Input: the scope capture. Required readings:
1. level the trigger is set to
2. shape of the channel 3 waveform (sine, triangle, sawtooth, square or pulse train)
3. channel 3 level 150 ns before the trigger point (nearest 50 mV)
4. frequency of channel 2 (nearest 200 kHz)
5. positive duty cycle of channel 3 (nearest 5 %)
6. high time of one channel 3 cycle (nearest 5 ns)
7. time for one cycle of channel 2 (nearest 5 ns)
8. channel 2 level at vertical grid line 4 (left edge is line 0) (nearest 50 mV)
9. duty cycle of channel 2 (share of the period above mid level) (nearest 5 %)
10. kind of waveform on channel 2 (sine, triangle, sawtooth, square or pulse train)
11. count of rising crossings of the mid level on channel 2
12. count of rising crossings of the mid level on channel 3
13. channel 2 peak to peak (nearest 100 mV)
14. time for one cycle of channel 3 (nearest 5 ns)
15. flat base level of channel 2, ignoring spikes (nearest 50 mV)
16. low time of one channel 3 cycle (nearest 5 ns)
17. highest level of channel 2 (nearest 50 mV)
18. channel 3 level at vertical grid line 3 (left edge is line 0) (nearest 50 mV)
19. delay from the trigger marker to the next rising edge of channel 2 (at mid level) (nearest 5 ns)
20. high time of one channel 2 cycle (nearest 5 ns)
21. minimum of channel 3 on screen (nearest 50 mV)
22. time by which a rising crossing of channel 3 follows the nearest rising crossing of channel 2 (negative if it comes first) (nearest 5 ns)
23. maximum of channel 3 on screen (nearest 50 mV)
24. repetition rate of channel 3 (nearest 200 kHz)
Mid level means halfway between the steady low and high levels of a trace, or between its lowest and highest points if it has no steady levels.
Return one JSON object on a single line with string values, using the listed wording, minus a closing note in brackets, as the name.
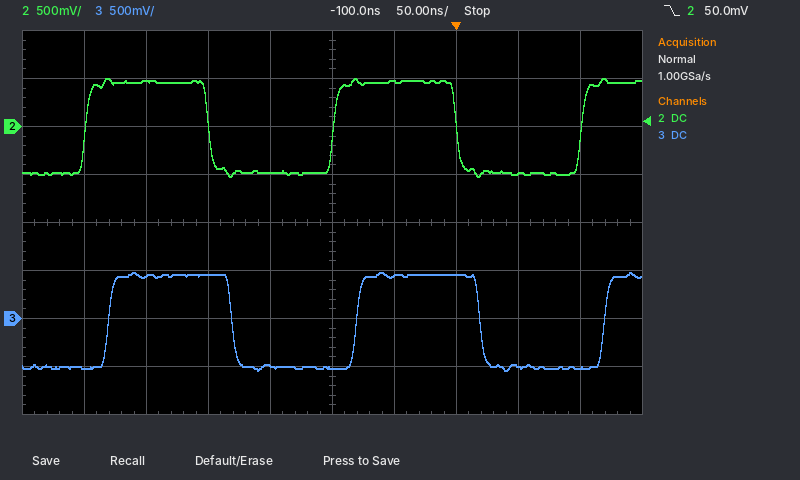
{"level the trigger is set to": "50.0 mV", "shape of the channel 3 waveform": "square", "channel 3 level 150 ns before the trigger point": "-500 mV", "frequency of channel 2": "5.0 MHz", "positive duty cycle of channel 3": "50 %", "high time of one channel 3 cycle": "100 ns", "time for one cycle of channel 2": "200 ns", "channel 2 level at vertical grid line 4 (left edge is line 0)": "-500 mV", "duty cycle of channel 2 (share of the period above mid level)": "50 %", "kind of waveform on channel 2": "square", "count of rising crossings of the mid level on channel 2": "3", "count of rising crossings of the mid level on channel 3": "3", "channel 2 peak to peak": "1.00 V", "time for one cycle of channel 3": "200 ns", "flat base level of channel 2, ignoring spikes": "-500 mV", "low time of one channel 3 cycle": "100 ns", "highest level of channel 2": "500 mV", "channel 3 level at vertical grid line 3 (left edge is line 0)": "450 mV", "delay from the trigger marker to the next rising edge of channel 2 (at mid level)": "100 ns", "high time of one channel 2 cycle": "100 ns", "minimum of channel 3 on screen": "-550 mV", "time by which a rising crossing of channel 3 follows the nearest rising crossing of channel 2 (negative if it comes first)": "+20 ns", "maximum of channel 3 on screen": "500 mV", "repetition rate of channel 3": "5.0 MHz"}
